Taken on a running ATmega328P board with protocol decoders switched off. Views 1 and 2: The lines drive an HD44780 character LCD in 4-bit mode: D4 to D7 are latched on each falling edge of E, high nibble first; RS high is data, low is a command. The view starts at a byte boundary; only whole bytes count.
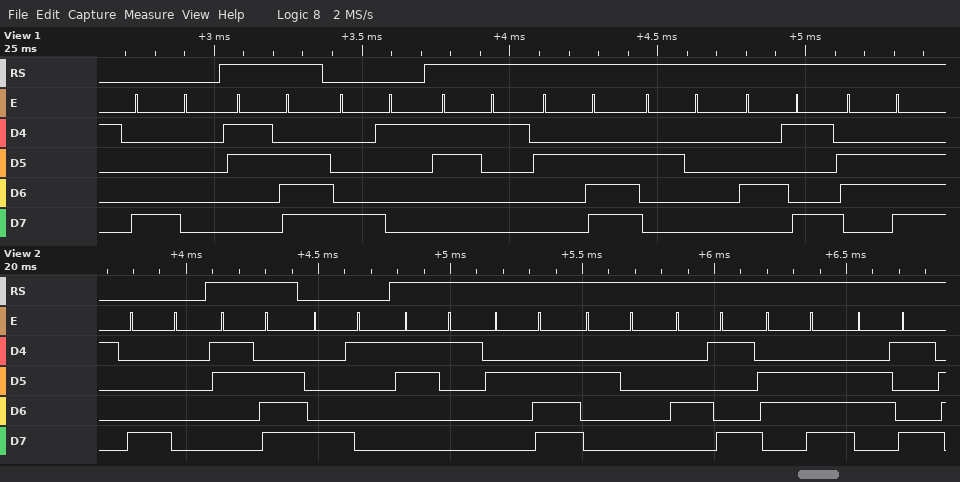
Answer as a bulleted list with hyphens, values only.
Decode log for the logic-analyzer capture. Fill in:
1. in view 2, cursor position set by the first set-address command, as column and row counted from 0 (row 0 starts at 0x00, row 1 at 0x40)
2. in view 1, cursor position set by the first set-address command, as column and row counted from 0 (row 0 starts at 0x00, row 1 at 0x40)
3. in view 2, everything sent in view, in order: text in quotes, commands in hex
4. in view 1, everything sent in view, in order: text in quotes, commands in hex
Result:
- column 0, row 0
- column 0, row 0
- 0x80 ">" 0x81 "1. Ini"
- 0x80 ">" 0x81 "1. In"
